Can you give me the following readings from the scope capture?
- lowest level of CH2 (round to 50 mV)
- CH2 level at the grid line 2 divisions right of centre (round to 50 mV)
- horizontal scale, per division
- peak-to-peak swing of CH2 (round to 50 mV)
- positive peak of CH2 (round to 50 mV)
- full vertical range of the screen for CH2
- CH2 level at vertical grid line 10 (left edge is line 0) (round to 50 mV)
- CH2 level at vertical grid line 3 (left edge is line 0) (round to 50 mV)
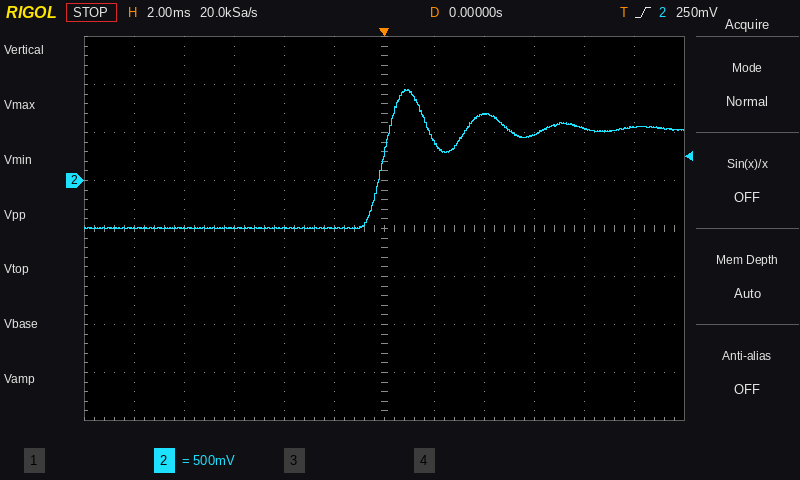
-500 mV
700 mV
2 ms
1.45 V
950 mV
4 V
550 mV
-500 mV
